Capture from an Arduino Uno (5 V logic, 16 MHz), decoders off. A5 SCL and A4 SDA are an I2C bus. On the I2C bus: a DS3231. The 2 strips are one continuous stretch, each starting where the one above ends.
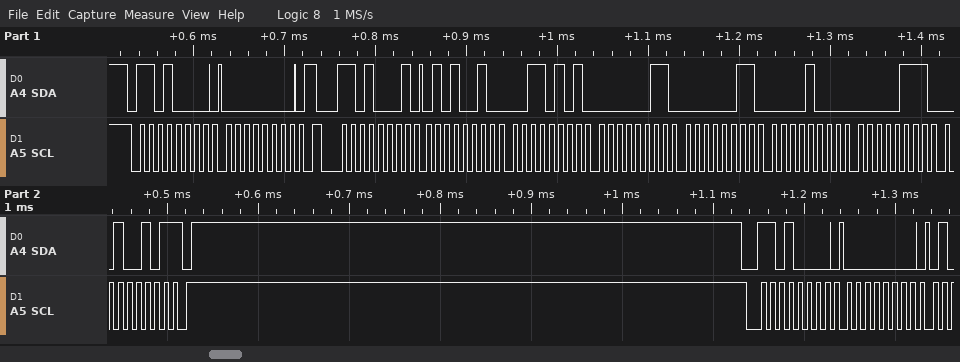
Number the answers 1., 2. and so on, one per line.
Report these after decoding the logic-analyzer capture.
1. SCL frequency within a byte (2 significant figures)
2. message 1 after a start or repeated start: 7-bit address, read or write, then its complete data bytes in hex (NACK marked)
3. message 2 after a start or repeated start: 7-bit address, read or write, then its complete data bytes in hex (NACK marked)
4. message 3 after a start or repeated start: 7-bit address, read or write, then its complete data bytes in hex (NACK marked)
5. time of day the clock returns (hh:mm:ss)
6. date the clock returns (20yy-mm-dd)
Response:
1. 100 kHz
2. 0x68 write: 00
3. 0x68 read: 52 35 03 03 08 07 25 NACK
4. 0x68 write: 00
5. 03:35:52
6. 2025-07-08
